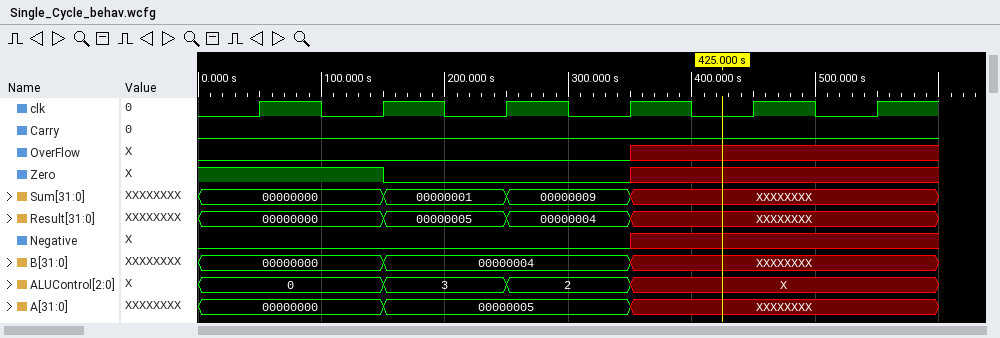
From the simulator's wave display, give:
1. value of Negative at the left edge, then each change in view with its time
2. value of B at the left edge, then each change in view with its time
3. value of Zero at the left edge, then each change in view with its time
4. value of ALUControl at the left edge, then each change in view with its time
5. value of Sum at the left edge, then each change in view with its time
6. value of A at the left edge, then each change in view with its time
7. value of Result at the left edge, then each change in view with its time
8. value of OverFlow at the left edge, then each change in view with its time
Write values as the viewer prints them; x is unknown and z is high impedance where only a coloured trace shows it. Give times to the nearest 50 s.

0, x at 350 s
00000000, 00000004 at 150 s, XXXXXXXX at 350 s
1, 0 at 150 s, x at 350 s
0, 3 at 150 s, 2 at 250 s, X at 350 s
00000000, 00000001 at 150 s, 00000009 at 250 s, XXXXXXXX at 350 s
00000000, 00000005 at 150 s, XXXXXXXX at 350 s
00000000, 00000005 at 150 s, 00000004 at 250 s, XXXXXXXX at 350 s
0, x at 350 s
